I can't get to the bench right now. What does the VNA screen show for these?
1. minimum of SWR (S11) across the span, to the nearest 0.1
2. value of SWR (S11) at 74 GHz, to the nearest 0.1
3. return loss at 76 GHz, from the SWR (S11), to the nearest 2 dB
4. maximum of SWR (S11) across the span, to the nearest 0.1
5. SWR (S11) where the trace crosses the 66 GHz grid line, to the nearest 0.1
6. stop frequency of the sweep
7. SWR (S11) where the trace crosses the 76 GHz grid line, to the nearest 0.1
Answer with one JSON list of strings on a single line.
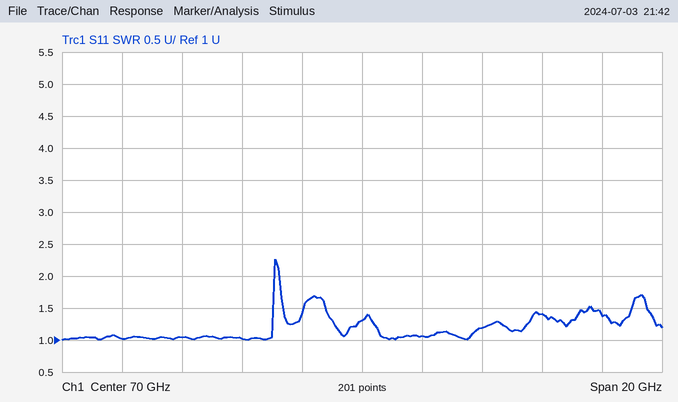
["1.0", "1.2", "16 dB", "2.3", "1.0", "80 GHz", "1.4"]
